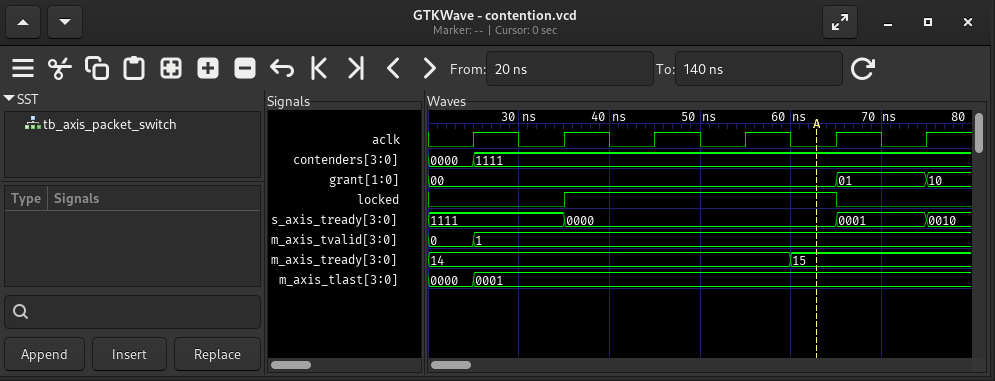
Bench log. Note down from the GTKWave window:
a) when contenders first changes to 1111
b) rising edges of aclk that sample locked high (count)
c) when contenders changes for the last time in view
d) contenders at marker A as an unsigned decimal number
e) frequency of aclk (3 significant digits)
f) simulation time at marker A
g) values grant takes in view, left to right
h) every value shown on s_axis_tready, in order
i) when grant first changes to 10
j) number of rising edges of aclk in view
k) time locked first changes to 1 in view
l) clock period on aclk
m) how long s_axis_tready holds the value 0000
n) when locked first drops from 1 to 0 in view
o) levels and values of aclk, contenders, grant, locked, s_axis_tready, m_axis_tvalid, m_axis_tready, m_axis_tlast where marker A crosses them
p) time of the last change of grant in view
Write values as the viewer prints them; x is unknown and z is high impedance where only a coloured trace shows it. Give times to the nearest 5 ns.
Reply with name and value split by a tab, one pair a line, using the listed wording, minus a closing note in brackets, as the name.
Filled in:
when contenders first changes to 1111	25 ns
rising edges of aclk that sample locked high	3
when contenders changes for the last time in view	25 ns
contenders at marker A as an unsigned decimal number	15
frequency of aclk	100 MHz
simulation time at marker A	65 ns
values grant takes in view, left to right	00, 01, 10
every value shown on s_axis_tready, in order	1111, 0000, 0001, 0010
when grant first changes to 10	75 ns
number of rising edges of aclk in view	6
time locked first changes to 1 in view	35 ns
clock period on aclk	10 ns
how long s_axis_tready holds the value 0000	30 ns
when locked first drops from 1 to 0 in view	65 ns
levels and values of aclk, contenders, grant, locked, s_axis_tready, m_axis_tvalid, m_axis_tready, m_axis_tlast where marker A crosses them	aclk=0, contenders=1111, grant=00, locked=1, s_axis_tready=0000, m_axis_tvalid=1, m_axis_tready=15, m_axis_tlast=0001
time of the last change of grant in view	75 ns
